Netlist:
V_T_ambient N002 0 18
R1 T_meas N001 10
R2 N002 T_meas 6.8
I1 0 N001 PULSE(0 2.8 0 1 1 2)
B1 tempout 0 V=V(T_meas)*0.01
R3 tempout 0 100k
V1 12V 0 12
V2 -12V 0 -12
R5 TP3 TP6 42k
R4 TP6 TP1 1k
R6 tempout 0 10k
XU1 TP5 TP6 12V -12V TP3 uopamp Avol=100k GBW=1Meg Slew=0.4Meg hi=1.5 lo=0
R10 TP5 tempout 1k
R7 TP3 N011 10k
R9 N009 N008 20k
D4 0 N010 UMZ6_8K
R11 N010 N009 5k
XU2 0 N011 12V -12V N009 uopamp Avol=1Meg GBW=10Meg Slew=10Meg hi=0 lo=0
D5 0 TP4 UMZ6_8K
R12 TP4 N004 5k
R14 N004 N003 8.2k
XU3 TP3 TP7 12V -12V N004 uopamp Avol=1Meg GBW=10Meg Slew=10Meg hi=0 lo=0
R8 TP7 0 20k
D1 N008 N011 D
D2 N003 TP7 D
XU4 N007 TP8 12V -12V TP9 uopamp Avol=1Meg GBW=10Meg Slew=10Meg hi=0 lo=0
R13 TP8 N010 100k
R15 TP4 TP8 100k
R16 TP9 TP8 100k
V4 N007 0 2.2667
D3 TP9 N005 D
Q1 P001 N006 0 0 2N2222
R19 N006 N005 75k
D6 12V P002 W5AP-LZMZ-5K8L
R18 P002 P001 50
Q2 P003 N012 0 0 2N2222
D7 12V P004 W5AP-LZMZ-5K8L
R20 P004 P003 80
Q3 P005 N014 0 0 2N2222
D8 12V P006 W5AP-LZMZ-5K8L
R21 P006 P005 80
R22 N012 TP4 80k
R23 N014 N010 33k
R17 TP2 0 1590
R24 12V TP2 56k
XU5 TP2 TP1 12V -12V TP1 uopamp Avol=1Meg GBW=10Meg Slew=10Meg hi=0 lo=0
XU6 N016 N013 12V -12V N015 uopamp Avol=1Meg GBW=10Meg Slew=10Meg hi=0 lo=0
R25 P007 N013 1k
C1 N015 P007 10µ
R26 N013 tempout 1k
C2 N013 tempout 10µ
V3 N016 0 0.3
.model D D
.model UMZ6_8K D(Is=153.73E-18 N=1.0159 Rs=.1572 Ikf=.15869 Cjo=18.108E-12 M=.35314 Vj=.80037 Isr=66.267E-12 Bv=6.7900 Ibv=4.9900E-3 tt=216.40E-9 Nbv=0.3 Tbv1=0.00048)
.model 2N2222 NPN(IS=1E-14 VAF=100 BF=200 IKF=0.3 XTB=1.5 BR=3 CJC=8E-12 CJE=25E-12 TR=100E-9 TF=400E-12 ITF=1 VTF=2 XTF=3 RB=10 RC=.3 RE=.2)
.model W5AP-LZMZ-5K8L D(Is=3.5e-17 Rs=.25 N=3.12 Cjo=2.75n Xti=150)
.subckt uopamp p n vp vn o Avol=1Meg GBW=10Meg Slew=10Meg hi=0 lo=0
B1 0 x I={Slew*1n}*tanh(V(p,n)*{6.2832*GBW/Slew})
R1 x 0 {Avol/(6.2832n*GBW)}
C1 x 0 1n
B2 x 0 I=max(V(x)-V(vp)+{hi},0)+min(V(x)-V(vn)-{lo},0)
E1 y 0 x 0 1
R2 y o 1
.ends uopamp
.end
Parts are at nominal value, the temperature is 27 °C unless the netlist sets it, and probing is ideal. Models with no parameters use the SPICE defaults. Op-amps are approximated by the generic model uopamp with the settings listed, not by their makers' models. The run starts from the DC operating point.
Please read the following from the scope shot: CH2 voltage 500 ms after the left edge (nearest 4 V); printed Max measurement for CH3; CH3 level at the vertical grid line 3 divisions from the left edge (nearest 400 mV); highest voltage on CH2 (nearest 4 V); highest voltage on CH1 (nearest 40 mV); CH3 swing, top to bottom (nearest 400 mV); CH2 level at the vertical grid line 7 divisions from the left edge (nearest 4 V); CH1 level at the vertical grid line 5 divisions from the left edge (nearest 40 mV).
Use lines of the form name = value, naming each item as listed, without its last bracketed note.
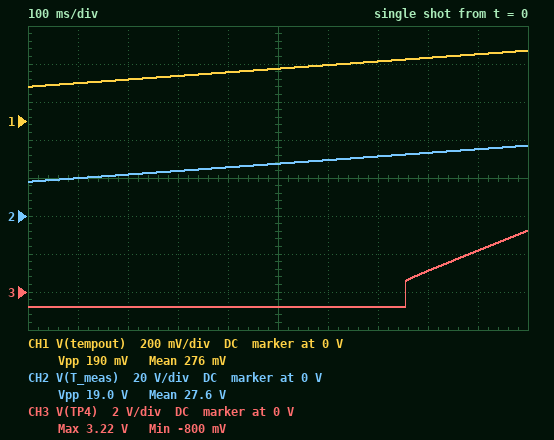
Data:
CH2 voltage 500 ms after the left edge = 28 V
printed Max measurement for CH3 = 3.22 V
CH3 level at the vertical grid line 3 divisions from the left edge = -800 mV
highest voltage on CH2 = 36 V
highest voltage on CH1 = 360 mV
CH3 swing, top to bottom = 4.0 V
CH2 level at the vertical grid line 7 divisions from the left edge = 32 V
CH1 level at the vertical grid line 5 divisions from the left edge = 280 mV
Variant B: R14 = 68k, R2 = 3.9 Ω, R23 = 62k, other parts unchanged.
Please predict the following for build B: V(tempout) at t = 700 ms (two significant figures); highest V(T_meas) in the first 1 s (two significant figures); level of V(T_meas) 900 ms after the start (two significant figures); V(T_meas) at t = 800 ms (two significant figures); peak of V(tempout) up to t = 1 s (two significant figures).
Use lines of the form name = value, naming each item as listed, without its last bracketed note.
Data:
V(tempout) at t = 700 ms = 260 mV
highest V(T_meas) in the first 1 s = 29 V
level of V(T_meas) 900 ms after the start = 28 V
V(T_meas) at t = 800 ms = 27 V
peak of V(tempout) up to t = 1 s = 290 mV
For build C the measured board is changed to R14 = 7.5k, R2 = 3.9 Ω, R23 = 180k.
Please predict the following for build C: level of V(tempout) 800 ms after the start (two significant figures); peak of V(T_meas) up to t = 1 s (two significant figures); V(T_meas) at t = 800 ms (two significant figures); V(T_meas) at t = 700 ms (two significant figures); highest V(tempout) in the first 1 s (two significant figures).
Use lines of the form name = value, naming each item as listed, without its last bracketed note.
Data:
level of V(tempout) 800 ms after the start = 270 mV
peak of V(T_meas) up to t = 1 s = 29 V
V(T_meas) at t = 800 ms = 27 V
V(T_meas) at t = 700 ms = 26 V
highest V(tempout) in the first 1 s = 290 mV
